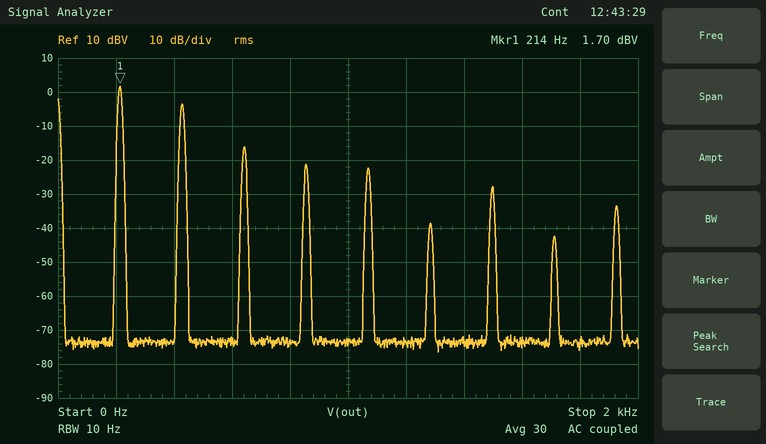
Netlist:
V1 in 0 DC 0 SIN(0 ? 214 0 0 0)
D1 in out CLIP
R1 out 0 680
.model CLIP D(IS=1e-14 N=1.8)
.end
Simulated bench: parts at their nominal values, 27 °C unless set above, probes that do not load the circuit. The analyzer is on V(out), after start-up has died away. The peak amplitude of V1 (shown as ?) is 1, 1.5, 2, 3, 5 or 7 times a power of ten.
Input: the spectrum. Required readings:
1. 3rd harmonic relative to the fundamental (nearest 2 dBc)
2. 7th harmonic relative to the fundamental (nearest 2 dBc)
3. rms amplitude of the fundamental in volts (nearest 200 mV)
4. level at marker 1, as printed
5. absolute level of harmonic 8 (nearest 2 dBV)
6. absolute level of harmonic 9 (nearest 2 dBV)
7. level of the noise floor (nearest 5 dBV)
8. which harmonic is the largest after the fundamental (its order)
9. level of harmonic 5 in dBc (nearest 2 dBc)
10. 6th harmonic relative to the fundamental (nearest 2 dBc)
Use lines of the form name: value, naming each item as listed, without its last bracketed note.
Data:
3rd harmonic relative to the fundamental: -18 dBc
7th harmonic relative to the fundamental: -30 dBc
rms amplitude of the fundamental in volts: 1.2 V
level at marker 1, as printed: 1.70 dBV
absolute level of harmonic 8: -42 dBV
absolute level of harmonic 9: -34 dBV
level of the noise floor: -75 dBV
which harmonic is the largest after the fundamental: 2
level of harmonic 5 in dBc: -24 dBc
6th harmonic relative to the fundamental: -40 dBc
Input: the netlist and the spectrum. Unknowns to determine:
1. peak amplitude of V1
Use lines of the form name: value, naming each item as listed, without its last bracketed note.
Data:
peak amplitude of V1: 5 V
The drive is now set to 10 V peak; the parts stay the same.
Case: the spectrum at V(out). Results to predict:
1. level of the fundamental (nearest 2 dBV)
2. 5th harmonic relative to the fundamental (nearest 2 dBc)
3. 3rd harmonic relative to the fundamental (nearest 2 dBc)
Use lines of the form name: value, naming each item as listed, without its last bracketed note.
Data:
level of the fundamental: 10 dBV
5th harmonic relative to the fundamental: -30 dBc
3rd harmonic relative to the fundamental: -24 dBc
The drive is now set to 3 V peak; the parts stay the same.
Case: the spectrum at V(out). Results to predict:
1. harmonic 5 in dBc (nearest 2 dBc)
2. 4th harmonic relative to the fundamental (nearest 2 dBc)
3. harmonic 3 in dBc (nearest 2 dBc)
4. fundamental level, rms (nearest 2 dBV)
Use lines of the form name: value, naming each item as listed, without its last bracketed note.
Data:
harmonic 5 in dBc: -22 dBc
4th harmonic relative to the fundamental: -36 dBc
harmonic 3 in dBc: -12 dBc
fundamental level, rms: -6 dBV
